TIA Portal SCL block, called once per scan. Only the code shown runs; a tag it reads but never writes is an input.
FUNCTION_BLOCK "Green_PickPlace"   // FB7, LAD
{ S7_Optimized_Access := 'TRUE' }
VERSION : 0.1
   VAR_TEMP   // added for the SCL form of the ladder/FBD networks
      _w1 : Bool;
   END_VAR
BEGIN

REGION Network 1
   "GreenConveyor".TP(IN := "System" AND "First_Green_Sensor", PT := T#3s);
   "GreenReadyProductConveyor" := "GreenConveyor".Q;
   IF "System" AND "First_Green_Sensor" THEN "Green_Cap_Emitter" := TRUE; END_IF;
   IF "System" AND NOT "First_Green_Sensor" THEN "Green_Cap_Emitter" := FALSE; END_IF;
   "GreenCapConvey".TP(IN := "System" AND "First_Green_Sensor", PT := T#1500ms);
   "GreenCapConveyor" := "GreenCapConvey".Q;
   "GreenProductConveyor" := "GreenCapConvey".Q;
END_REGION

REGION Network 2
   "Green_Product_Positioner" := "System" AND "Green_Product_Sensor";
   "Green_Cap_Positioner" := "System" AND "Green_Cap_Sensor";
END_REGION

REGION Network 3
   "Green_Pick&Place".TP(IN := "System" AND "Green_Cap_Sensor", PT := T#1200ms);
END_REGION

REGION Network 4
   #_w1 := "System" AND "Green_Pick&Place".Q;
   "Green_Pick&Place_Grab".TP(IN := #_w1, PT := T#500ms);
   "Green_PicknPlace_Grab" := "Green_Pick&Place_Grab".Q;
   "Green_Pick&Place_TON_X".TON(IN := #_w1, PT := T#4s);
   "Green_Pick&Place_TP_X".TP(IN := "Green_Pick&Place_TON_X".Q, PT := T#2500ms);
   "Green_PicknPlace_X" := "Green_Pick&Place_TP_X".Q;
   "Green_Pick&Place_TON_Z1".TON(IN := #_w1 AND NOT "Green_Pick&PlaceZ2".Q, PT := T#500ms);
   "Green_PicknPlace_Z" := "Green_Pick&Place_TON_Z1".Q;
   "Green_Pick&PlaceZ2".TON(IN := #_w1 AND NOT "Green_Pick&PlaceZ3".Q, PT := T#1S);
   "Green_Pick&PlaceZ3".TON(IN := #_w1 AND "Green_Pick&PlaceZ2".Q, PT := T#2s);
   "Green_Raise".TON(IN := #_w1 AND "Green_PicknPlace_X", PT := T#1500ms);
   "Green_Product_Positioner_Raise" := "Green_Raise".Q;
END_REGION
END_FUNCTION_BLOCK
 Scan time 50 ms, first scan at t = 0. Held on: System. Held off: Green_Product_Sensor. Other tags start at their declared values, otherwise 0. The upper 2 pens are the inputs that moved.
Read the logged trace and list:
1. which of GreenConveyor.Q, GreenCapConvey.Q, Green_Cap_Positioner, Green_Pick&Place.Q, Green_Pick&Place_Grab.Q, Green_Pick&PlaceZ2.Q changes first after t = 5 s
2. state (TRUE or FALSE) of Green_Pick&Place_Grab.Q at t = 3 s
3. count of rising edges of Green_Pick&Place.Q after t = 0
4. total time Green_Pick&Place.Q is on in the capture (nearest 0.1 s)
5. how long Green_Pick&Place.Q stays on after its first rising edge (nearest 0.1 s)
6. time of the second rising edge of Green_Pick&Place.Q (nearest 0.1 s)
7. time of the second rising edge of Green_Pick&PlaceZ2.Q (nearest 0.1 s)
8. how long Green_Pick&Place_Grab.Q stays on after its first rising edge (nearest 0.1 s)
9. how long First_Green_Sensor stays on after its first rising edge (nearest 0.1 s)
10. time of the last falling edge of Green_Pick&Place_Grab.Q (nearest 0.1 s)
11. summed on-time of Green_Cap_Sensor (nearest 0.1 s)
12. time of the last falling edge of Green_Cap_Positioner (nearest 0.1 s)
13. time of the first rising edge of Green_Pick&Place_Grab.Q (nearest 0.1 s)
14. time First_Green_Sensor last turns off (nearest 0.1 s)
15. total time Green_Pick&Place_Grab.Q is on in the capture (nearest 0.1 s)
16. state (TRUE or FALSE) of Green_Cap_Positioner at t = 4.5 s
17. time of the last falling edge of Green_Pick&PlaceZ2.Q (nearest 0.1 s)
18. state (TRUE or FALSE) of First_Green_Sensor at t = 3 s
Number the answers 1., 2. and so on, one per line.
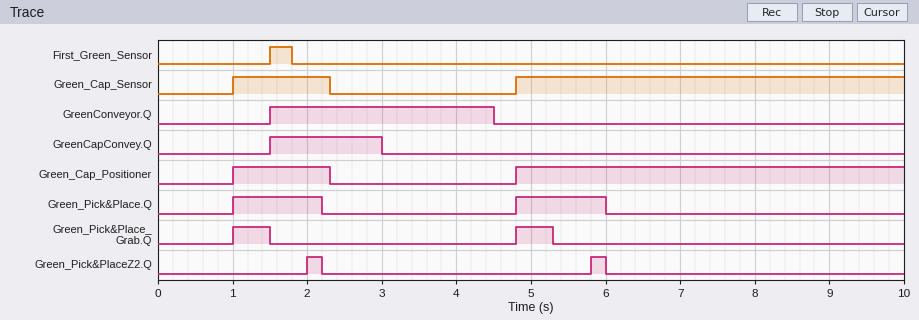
1. Green_Pick&Place_Grab.Q
2. FALSE
3. 2
4. 2.4 s
5. 1.2 s
6. 4.8 s
7. 5.8 s
8. 0.5 s
9. 0.3 s
10. 5.3 s
11. 6.5 s
12. 2.3 s
13. 1.0 s
14. 1.8 s
15. 1.0 s
16. FALSE
17. 6.0 s
18. FALSE
